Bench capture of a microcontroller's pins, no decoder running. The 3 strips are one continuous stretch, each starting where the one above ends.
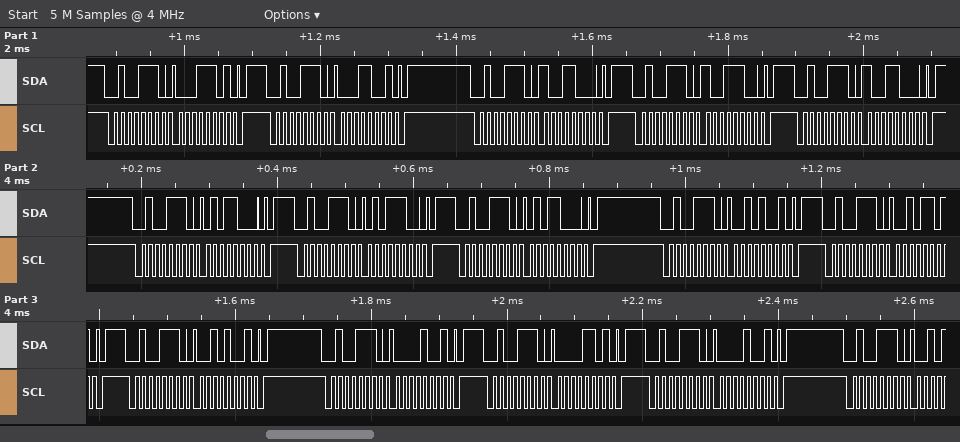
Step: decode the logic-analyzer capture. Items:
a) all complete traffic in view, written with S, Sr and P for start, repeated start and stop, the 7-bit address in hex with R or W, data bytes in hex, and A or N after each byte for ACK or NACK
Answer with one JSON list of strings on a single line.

["S 27W A 1D A P S 27W A 19 A P S 27W A 98 A P S 27W A 9C A P S 27W A 98 A P S 27W A 58 A P S 27W A 5C A P S 27W A 58 A P S 27W A 29 A P S 27W A 2D A P S 27W A 29 A P S 27W A 09 A P S 27W A 0D A P S 27W A 09 A P S 27W A"]
